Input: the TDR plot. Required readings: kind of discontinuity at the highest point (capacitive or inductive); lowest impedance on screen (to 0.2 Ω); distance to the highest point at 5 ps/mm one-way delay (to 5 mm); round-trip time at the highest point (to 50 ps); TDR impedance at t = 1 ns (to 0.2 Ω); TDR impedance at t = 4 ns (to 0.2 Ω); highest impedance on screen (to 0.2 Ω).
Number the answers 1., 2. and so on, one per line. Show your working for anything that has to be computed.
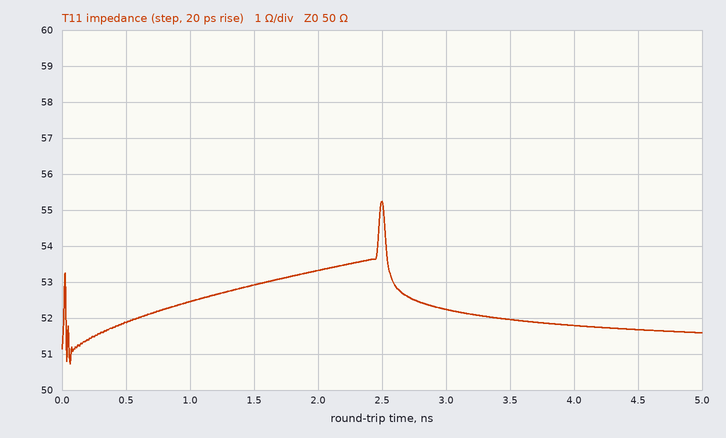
1. inductive
2. 50.8 Ω
3. 2.50 ns / 2 / 5 ps/mm ≈ 250 mm
4. 2.50 ns
5. 52.4 Ω
6. 51.8 Ω
7. 55.2 Ω
